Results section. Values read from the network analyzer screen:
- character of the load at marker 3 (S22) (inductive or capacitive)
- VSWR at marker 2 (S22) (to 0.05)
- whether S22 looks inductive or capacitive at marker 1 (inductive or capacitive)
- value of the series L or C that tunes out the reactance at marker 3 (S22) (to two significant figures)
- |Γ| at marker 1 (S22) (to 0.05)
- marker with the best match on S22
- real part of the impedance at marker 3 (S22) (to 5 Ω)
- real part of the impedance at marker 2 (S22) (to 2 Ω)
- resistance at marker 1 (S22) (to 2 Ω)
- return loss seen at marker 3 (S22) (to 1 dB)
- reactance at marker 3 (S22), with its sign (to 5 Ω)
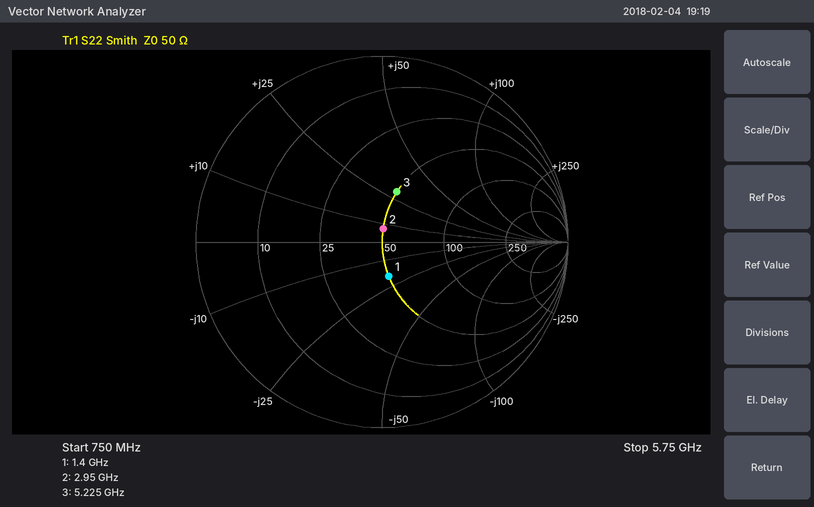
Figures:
inductive
1.15
capacitive
1.0 pF
0.20
marker 2
50 Ω
50 Ω
50 Ω
11 dB
+30 Ω
